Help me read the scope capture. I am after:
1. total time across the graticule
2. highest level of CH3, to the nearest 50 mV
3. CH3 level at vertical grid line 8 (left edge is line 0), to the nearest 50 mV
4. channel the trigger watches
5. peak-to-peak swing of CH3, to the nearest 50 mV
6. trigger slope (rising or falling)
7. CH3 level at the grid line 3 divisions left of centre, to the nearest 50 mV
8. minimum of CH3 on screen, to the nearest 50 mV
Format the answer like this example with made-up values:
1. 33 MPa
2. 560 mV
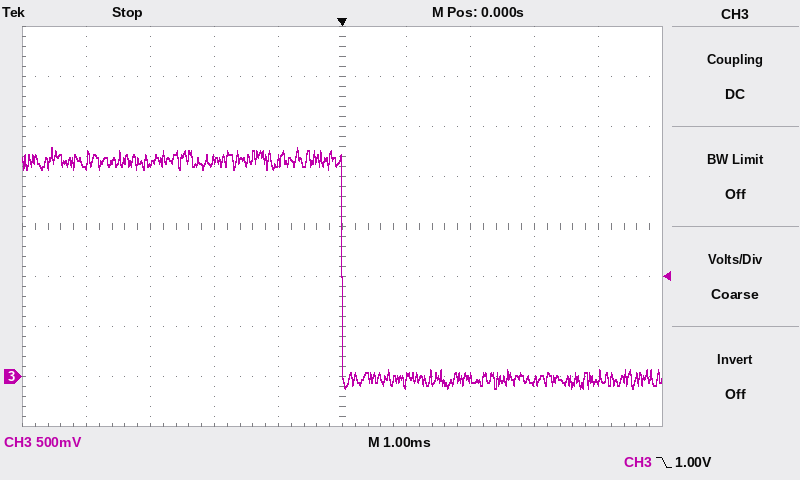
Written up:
1. 10 ms
2. 2.30 V
3. -50 mV
4. CH3
5. 2.40 V
6. falling
7. 2.15 V
8. -100 mV
